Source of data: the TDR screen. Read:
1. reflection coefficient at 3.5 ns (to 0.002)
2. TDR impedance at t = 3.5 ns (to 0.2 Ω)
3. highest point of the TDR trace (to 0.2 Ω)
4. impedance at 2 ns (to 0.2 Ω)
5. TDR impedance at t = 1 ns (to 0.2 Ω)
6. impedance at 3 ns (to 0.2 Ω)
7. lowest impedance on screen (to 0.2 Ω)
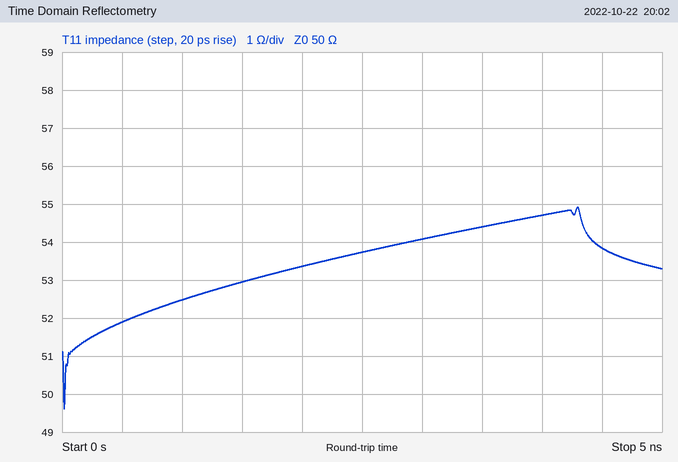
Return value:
+0.042
54.4 Ω
55.0 Ω
53.4 Ω
52.4 Ω
54.0 Ω
49.6 Ω
